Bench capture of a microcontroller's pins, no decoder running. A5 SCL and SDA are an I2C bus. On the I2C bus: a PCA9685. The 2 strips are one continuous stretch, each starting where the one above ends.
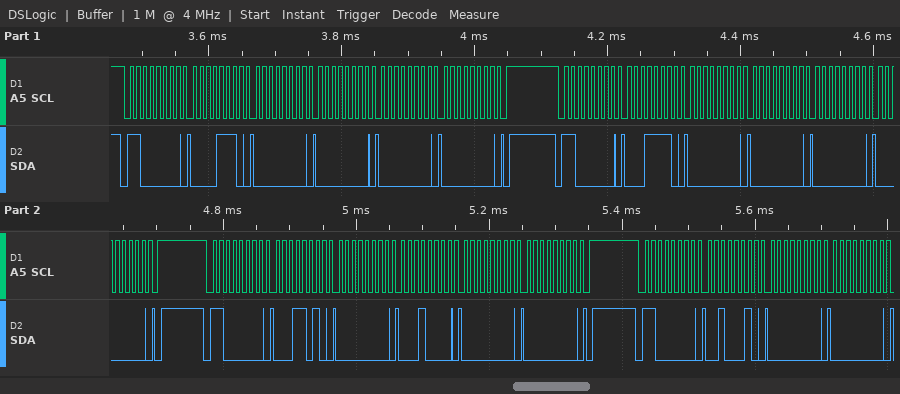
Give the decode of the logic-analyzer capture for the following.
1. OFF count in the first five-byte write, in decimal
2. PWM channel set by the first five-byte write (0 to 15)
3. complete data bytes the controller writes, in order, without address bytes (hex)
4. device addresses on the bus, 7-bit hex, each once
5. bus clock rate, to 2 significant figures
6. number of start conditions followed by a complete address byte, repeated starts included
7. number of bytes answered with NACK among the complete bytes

0
2
0E 00 00 00 00 1E 00 00 00 00 1A 00 10 00 00 22 00 00
0x60
100 kHz
4
0
